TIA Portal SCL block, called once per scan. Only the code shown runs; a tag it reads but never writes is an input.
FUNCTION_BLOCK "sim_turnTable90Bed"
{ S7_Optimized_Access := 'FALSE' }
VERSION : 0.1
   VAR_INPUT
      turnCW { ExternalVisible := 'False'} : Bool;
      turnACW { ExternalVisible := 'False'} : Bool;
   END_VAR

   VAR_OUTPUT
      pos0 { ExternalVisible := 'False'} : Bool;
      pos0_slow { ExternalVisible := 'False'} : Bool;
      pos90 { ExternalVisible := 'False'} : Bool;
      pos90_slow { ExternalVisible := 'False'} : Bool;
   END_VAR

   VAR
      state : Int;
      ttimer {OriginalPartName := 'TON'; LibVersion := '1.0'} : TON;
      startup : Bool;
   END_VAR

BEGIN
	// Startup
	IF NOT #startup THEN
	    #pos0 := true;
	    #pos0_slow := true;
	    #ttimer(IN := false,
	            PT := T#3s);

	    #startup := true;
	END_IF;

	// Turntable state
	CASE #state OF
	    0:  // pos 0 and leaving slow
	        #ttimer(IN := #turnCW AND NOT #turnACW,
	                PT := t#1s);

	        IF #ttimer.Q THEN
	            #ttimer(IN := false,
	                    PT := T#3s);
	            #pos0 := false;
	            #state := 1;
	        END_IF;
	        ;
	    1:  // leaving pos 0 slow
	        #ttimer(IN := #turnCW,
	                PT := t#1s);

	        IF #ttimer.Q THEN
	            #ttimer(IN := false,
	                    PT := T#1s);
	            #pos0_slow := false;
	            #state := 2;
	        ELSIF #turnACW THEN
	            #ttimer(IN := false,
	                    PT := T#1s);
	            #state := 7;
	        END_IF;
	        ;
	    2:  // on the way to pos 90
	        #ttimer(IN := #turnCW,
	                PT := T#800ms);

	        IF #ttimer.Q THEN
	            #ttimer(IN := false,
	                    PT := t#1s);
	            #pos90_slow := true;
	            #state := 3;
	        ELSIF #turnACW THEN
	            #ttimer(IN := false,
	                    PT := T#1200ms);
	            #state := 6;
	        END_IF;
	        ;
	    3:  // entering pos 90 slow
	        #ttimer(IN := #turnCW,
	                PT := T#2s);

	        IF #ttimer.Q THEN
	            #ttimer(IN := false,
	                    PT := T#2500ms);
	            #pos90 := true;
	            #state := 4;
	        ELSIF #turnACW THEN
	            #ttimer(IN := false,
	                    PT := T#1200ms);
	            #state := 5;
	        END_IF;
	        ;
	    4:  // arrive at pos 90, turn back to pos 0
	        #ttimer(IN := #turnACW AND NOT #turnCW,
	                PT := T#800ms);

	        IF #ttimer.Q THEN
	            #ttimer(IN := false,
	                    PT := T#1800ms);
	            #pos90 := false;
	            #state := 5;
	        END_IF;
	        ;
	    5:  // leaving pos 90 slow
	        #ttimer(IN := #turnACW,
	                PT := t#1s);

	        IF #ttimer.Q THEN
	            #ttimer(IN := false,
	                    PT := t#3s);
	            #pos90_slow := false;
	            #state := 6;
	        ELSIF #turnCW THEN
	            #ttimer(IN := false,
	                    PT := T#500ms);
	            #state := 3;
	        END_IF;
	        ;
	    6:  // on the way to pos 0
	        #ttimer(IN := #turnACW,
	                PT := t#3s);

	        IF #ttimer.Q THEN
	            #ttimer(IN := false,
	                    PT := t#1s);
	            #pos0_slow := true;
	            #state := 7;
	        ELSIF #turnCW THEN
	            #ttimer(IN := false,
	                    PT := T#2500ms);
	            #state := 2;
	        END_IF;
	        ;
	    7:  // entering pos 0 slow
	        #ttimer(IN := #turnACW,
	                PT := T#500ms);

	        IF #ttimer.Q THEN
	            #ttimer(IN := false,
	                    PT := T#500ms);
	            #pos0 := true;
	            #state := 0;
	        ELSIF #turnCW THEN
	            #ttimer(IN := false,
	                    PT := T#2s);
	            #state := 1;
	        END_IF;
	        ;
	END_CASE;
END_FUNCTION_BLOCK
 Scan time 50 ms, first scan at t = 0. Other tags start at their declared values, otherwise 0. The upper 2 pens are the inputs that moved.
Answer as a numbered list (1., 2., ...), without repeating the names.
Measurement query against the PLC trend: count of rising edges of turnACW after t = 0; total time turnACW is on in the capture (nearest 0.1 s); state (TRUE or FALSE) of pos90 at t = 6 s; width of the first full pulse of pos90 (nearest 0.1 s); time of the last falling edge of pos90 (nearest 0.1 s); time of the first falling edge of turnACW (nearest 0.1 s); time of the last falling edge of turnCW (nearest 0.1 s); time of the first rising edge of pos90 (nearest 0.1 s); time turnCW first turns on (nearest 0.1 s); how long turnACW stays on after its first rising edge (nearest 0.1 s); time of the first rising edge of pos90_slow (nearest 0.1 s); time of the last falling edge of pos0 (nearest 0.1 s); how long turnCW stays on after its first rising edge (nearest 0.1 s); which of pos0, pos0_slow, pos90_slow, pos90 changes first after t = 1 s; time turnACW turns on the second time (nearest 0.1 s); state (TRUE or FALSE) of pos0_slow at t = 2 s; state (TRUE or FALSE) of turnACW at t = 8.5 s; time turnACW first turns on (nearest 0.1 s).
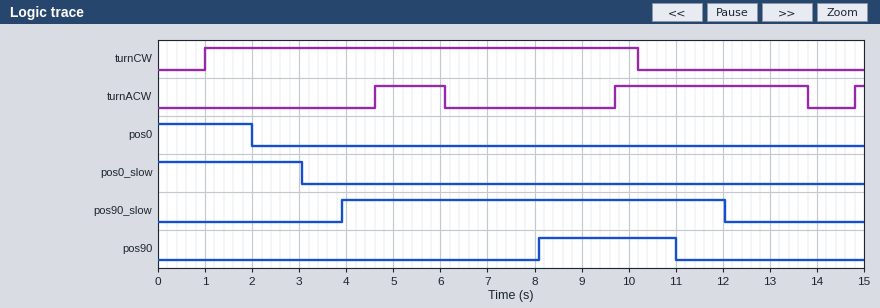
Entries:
1. 3
2. 5.8 s
3. FALSE
4. 2.9 s
5. 11.0 s
6. 6.1 s
7. 10.2 s
8. 8.1 s
9. 1.0 s
10. 1.5 s
11. 3.9 s
12. 2.0 s
13. 9.2 s
14. pos0
15. 9.7 s
16. TRUE
17. FALSE
18. 4.6 s
